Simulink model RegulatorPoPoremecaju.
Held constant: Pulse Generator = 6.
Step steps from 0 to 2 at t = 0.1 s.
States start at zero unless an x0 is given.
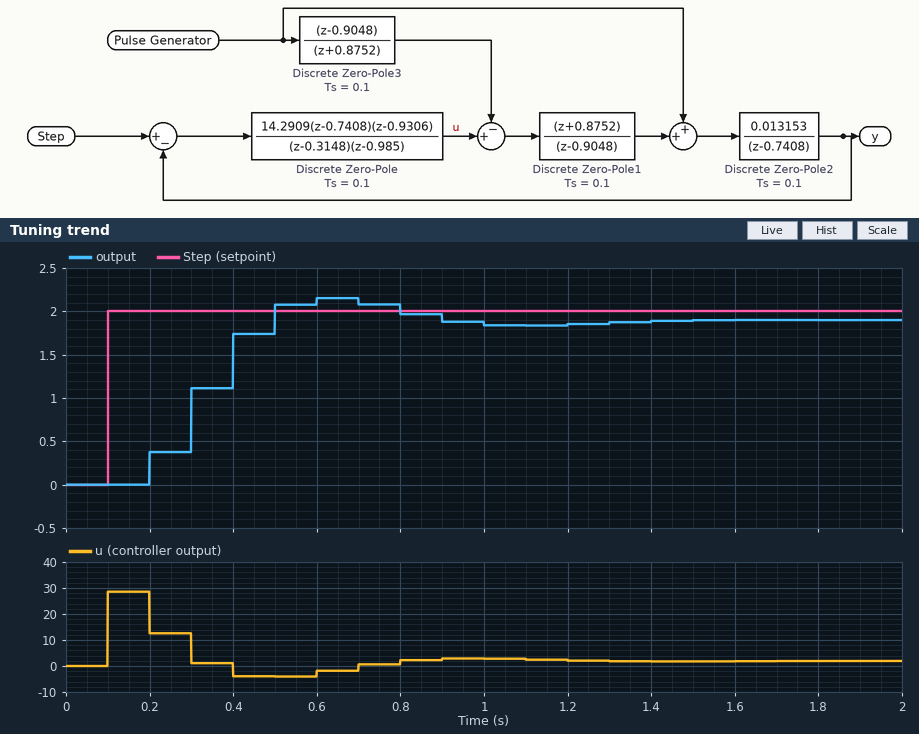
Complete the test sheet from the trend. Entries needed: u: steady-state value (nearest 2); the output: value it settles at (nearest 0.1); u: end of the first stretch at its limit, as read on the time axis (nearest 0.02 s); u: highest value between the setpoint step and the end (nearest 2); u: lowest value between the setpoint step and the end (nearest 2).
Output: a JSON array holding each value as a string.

["2", "1.9", "0.20 s", "28", "-4"]
